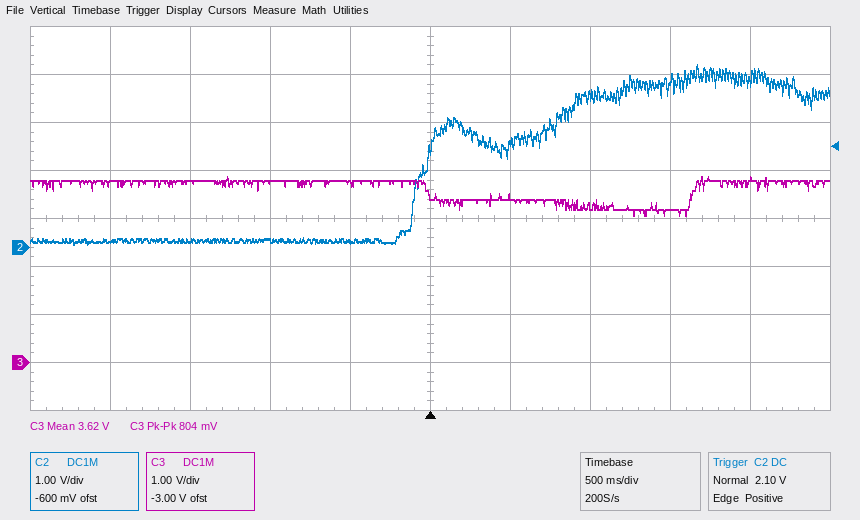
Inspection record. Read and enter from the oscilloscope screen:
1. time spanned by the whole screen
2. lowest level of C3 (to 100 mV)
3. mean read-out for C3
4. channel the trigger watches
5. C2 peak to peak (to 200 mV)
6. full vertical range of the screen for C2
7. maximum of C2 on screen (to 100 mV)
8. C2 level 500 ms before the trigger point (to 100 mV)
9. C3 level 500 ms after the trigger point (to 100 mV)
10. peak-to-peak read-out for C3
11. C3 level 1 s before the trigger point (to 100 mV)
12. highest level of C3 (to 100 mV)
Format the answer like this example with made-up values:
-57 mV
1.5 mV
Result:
5 s
3.1 V
3.62 V
C2
3.8 V
8 V
3.8 V
100 mV
3.5 V
804 mV
3.8 V
3.9 V
